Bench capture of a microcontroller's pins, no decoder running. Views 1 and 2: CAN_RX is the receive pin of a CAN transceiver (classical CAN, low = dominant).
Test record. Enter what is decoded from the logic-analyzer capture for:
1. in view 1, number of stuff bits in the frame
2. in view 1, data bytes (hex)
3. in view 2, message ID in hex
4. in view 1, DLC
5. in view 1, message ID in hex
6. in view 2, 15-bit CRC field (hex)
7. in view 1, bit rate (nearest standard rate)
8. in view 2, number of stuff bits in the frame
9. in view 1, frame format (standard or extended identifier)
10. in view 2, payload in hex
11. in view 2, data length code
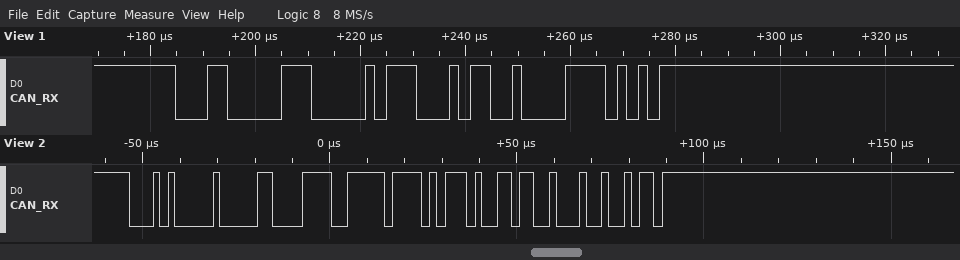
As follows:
2
C5
0x140
1
0x183
0x1125
500 kbit/s
3
standard
3C FF AE 9B
4
